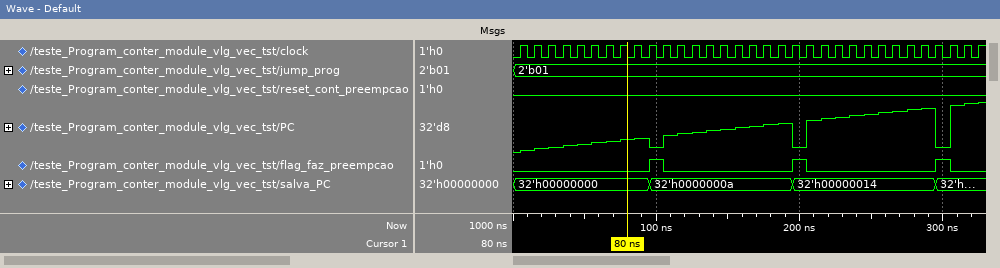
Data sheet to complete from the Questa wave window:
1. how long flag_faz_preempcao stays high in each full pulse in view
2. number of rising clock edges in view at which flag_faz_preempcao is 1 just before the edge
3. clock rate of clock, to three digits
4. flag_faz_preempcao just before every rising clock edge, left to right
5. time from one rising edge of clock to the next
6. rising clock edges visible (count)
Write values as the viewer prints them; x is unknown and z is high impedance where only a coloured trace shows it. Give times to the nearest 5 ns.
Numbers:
10 ns, 10 ns, 10 ns
3
100 MHz
0 0 0 0 0 0 0 0 0 0 1 0 0 0 0 0 0 0 0 0 1 0 0 0 0 0 0 0 0 0 1 0 0
10 ns
33
